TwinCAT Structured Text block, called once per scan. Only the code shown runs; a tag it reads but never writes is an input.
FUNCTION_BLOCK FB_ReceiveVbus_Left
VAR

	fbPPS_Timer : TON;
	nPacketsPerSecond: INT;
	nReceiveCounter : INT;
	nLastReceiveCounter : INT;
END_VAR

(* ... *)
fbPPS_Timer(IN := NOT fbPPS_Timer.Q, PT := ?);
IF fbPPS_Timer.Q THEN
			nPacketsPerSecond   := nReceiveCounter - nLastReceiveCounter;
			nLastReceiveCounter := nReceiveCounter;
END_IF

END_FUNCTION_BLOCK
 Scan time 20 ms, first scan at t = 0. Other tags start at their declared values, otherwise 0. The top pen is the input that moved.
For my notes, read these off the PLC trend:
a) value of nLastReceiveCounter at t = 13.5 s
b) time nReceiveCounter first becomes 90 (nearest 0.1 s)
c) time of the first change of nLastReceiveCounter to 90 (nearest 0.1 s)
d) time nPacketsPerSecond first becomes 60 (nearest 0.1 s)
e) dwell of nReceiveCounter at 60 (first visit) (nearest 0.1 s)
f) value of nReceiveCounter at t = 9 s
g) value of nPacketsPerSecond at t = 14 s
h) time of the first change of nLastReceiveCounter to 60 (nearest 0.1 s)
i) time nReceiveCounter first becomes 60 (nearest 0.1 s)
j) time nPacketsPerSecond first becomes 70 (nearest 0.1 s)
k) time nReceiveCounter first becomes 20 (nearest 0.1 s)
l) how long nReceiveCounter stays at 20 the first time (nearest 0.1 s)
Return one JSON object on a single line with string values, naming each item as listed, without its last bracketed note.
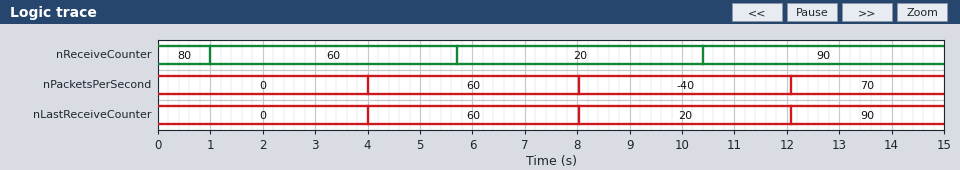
{"value of nLastReceiveCounter at t = 13.5 s": "90", "time nReceiveCounter first becomes 90": "10.4 s", "time of the first change of nLastReceiveCounter to 90": "12.1 s", "time nPacketsPerSecond first becomes 60": "4.0 s", "dwell of nReceiveCounter at 60 (first visit)": "4.7 s", "value of nReceiveCounter at t = 9 s": "20", "value of nPacketsPerSecond at t = 14 s": "70", "time of the first change of nLastReceiveCounter to 60": "4.0 s", "time nReceiveCounter first becomes 60": "1.0 s", "time nPacketsPerSecond first becomes 70": "12.1 s", "time nReceiveCounter first becomes 20": "5.7 s", "how long nReceiveCounter stays at 20 the first time": "4.7 s"}
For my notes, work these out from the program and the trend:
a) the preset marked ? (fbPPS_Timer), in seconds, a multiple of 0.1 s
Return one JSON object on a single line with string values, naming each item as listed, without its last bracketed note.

{"the preset marked ? (fbPPS_Timer), in seconds, a multiple of 0.1 s": "4.0 s"}
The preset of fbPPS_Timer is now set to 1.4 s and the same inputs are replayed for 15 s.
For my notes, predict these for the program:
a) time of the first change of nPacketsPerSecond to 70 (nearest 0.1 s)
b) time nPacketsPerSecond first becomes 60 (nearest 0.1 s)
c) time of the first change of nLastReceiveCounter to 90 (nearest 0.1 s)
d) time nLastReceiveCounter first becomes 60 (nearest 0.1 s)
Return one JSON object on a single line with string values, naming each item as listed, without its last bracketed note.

{"time of the first change of nPacketsPerSecond to 70": "11.5 s", "time nPacketsPerSecond first becomes 60": "1.4 s", "time of the first change of nLastReceiveCounter to 90": "11.5 s", "time nLastReceiveCounter first becomes 60": "1.4 s"}
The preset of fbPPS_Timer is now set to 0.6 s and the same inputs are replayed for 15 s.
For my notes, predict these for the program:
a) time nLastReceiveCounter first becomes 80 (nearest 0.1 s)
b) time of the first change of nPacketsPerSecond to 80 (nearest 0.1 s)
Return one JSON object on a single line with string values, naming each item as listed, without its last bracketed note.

{"time nLastReceiveCounter first becomes 80": "0.6 s", "time of the first change of nPacketsPerSecond to 80": "0.6 s"}
